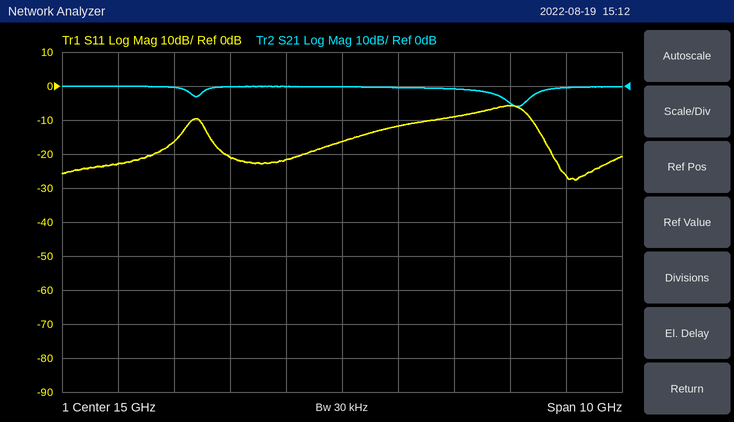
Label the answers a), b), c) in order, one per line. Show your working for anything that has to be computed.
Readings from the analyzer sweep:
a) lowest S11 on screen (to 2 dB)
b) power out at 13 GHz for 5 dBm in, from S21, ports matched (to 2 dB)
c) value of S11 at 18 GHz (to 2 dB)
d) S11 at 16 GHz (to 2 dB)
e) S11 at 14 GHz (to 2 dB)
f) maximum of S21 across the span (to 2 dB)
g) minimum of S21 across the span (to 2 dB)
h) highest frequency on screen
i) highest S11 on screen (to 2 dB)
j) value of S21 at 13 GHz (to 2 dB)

a) -28 dB
b) 5 dBm + (0 dB) = 4 dBm
c) -6 dB
d) -12 dB
e) -22 dB
f) 0 dB
g) -6 dB
h) 20 GHz
i) -6 dB
j) 0 dB
